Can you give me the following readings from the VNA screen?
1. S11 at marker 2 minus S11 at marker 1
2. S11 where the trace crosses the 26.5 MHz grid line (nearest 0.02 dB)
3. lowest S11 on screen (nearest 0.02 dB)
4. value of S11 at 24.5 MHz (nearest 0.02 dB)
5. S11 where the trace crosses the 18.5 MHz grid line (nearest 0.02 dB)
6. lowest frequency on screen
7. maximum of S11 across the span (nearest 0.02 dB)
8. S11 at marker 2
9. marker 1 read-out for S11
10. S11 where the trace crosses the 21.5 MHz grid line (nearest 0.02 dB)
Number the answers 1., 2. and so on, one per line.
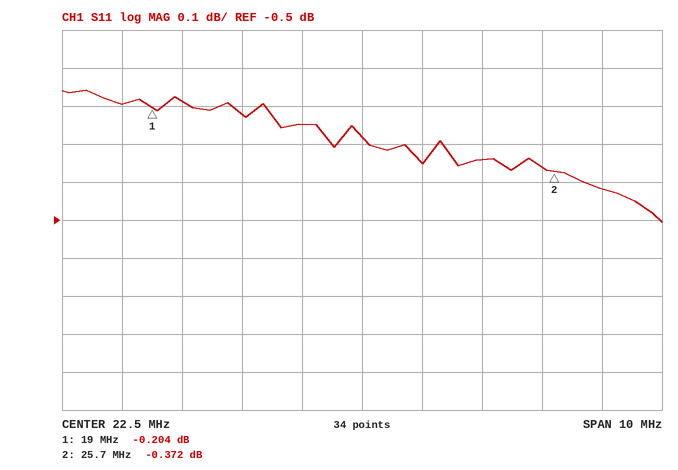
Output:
1. -0.168 dB
2. -0.42 dB
3. -0.50 dB
4. -0.34 dB
5. -0.20 dB
6. 17.5 MHz
7. -0.16 dB
8. -0.372 dB
9. -0.204 dB
10. -0.24 dB
